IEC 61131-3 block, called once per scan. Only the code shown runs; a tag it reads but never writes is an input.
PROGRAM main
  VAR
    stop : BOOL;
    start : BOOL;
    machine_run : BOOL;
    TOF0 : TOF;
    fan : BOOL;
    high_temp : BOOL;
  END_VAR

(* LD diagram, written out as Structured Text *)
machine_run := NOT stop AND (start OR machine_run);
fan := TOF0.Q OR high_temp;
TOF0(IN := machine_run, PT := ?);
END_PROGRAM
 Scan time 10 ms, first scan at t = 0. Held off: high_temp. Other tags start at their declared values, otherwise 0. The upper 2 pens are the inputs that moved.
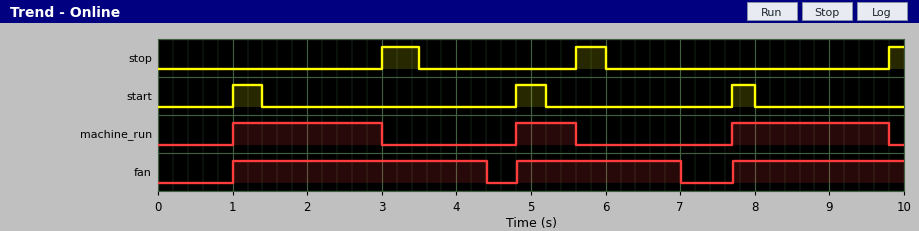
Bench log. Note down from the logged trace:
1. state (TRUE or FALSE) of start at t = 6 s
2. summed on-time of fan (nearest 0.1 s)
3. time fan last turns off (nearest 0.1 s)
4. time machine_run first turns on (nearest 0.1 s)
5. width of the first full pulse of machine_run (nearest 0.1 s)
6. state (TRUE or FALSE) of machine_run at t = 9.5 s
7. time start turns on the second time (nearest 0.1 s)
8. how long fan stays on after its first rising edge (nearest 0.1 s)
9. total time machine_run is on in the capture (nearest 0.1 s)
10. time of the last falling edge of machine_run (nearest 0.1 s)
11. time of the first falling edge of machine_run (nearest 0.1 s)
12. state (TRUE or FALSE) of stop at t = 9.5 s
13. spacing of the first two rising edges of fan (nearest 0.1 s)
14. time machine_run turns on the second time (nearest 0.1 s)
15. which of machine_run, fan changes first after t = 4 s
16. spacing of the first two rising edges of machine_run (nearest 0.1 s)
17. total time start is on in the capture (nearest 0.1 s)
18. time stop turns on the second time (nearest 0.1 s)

FALSE
7.9 s
7.0 s
1.0 s
2.0 s
TRUE
4.8 s
3.4 s
4.9 s
9.8 s
3.0 s
FALSE
3.8 s
4.8 s
fan
3.8 s
1.1 s
5.6 s
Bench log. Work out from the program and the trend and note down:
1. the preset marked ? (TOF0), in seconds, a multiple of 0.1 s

1.4 s
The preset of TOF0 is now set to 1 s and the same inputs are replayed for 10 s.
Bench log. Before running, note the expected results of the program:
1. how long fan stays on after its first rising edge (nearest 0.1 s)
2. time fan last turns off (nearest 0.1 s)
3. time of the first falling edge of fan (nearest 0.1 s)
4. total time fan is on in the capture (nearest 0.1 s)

3.0 s
6.6 s
4.0 s
7.1 s
